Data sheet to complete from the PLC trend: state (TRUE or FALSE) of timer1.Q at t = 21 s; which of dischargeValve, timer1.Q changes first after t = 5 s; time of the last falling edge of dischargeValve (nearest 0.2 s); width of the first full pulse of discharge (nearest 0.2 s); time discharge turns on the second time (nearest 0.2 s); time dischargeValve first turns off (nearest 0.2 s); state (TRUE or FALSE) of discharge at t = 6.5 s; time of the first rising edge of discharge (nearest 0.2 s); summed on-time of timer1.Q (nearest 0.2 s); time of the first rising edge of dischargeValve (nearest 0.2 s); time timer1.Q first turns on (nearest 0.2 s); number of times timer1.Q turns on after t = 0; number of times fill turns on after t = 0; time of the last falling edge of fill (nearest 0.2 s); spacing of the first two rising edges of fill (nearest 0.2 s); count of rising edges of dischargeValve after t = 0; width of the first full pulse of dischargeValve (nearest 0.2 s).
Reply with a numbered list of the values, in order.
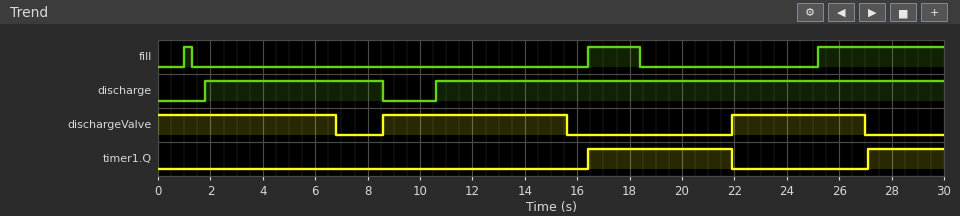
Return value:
1. TRUE
2. dischargeValve
3. 27.0 s
4. 6.8 s
5. 10.6 s
6. 6.8 s
7. TRUE
8. 1.8 s
9. 8.4 s
10. 8.6 s
11. 16.4 s
12. 2
13. 3
14. 18.4 s
15. 15.4 s
16. 2
17. 7.0 s
